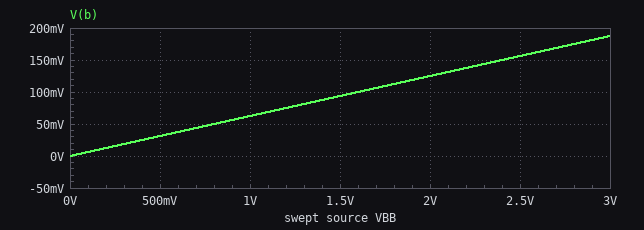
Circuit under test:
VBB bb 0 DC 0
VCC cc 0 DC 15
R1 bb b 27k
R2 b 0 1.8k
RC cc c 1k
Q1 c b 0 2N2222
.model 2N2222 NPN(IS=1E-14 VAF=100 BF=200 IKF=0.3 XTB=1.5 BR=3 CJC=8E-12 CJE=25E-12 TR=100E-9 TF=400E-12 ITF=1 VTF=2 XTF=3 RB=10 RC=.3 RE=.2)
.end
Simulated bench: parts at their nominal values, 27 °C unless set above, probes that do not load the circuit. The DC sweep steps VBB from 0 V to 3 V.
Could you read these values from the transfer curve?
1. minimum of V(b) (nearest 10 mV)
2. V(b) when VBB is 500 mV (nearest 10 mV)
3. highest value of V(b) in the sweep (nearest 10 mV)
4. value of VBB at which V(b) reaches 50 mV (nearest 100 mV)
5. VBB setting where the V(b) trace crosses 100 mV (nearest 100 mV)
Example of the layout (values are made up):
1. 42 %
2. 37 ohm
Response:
1. 0 V
2. 30 mV
3. 190 mV
4. 800 mV
5. 1.6 V
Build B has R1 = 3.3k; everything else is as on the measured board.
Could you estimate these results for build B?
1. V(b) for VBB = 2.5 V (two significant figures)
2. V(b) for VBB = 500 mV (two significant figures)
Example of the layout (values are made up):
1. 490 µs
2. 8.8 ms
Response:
1. 730 mV
2. 180 mV
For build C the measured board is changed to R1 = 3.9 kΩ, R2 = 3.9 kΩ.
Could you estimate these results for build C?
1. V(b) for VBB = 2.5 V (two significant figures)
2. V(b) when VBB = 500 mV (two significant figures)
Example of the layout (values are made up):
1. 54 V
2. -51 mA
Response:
1. 730 mV
2. 250 mV
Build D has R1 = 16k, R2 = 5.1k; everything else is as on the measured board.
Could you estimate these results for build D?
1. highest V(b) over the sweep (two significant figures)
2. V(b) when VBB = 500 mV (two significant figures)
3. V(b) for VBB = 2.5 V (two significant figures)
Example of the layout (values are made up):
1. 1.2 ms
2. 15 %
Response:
1. 680 mV
2. 120 mV
3. 600 mV
